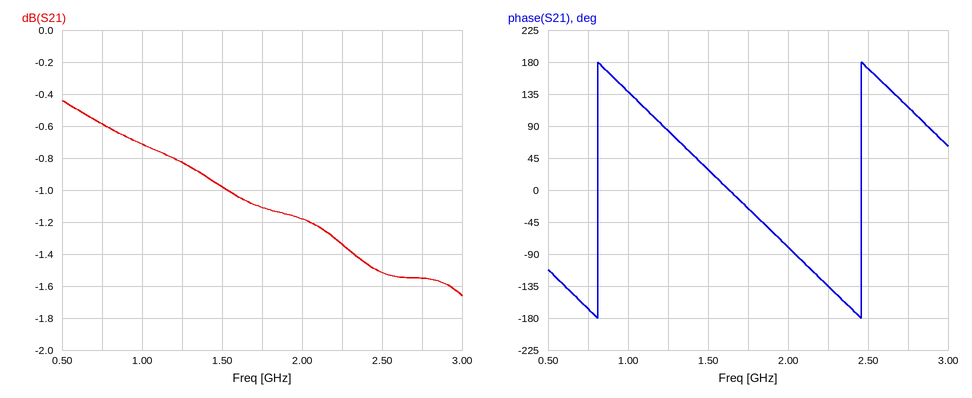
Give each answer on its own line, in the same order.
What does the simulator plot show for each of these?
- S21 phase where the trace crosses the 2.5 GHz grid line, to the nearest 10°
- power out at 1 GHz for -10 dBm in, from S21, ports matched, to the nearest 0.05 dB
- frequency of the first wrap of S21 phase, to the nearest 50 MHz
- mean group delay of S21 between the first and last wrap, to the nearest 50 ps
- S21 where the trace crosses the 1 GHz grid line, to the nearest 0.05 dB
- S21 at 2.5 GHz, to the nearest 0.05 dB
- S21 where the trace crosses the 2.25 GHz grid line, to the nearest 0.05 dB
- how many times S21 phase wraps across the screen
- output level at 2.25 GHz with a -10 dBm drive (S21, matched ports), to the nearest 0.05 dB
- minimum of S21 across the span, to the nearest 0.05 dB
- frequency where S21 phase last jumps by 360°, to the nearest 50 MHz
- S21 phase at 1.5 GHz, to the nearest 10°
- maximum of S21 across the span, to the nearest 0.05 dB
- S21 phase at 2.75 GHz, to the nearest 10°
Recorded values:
170°
-10.70 dBm
800 MHz
600 ps
-0.70 dB
-1.50 dB
-1.35 dB
2
-11.35 dBm
-1.65 dB
2.45 GHz
30°
-0.45 dB
120°
